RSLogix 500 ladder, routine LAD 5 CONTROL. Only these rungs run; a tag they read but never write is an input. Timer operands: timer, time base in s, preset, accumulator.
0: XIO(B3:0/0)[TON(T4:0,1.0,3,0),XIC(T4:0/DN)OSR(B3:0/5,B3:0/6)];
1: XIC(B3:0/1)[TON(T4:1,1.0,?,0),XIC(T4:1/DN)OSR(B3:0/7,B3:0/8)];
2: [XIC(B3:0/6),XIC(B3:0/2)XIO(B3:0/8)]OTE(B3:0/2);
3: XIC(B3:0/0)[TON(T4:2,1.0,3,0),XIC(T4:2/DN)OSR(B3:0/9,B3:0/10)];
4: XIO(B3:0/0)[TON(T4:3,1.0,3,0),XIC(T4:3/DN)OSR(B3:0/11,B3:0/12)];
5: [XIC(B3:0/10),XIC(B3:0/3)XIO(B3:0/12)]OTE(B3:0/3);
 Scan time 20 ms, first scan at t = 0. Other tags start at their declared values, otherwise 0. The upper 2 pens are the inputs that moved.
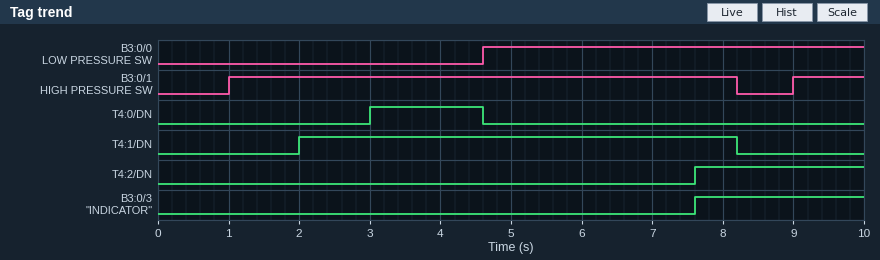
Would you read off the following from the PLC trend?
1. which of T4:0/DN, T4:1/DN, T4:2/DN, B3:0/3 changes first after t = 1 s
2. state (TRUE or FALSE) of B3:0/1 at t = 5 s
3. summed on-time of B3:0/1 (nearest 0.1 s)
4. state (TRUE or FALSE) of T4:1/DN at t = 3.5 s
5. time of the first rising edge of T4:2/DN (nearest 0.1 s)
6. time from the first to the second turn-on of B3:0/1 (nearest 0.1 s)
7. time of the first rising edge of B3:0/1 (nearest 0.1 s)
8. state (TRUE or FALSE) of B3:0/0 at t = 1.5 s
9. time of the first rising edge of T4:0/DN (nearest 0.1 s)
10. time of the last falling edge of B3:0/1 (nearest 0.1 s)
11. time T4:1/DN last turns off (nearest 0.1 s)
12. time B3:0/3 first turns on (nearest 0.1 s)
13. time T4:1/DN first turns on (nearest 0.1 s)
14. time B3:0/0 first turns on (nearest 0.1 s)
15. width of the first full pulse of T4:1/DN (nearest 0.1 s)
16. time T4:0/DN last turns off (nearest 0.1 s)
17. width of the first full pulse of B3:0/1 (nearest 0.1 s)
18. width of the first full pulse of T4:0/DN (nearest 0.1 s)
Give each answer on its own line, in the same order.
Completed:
T4:1/DN
TRUE
8.2 s
TRUE
7.6 s
8.0 s
1.0 s
FALSE
3.0 s
8.2 s
8.2 s
7.6 s
2.0 s
4.6 s
6.2 s
4.6 s
7.2 s
1.6 s
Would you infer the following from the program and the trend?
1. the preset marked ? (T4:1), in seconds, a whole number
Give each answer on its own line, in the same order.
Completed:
1 s
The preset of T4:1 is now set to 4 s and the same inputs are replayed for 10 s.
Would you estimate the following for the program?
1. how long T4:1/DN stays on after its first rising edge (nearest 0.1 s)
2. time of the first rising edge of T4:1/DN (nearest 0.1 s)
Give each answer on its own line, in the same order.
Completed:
3.2 s
5.0 s
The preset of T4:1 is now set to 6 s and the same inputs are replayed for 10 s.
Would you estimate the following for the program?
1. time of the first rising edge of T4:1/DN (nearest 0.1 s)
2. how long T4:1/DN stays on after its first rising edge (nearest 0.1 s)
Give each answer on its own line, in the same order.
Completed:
7.0 s
1.2 s
